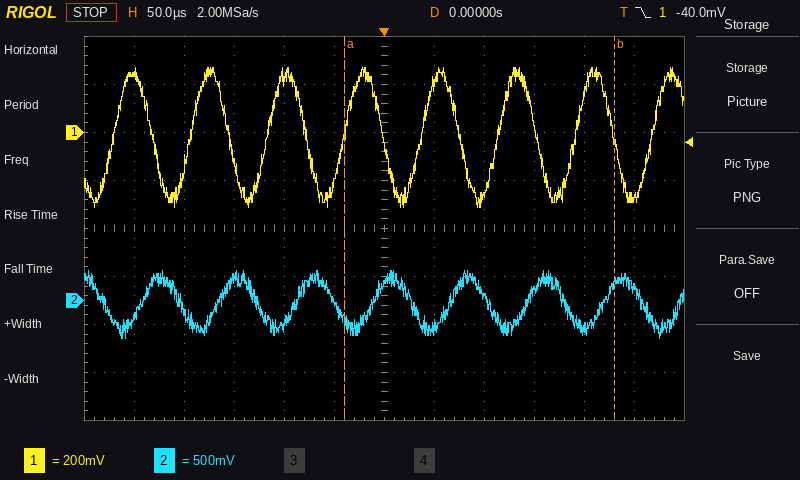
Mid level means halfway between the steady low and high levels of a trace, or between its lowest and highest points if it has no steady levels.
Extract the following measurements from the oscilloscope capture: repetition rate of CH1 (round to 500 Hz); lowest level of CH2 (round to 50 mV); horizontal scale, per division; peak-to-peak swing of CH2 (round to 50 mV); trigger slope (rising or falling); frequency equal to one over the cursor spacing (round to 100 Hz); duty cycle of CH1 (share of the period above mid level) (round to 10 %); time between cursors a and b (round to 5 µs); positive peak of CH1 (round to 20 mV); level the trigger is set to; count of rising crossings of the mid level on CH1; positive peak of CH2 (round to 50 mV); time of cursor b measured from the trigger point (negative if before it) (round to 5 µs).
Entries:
13.0 kHz
-400 mV
50 µs
700 mV
falling
3.7 kHz
50 %
270 µs
280 mV
-40.0 mV
8
300 mV
+230 µs
